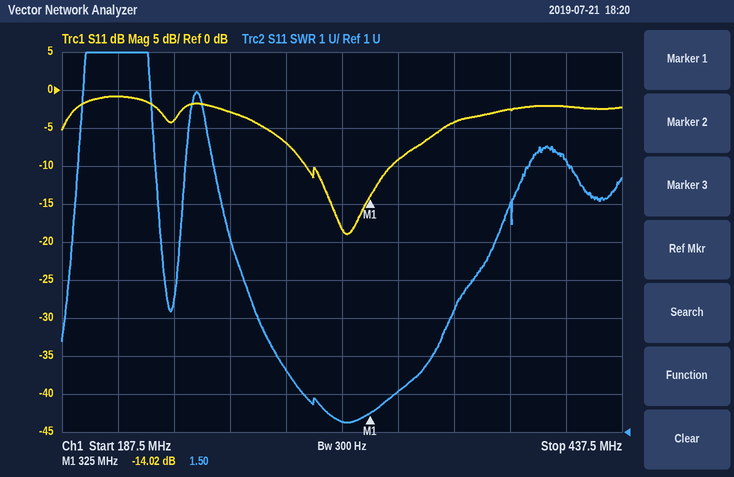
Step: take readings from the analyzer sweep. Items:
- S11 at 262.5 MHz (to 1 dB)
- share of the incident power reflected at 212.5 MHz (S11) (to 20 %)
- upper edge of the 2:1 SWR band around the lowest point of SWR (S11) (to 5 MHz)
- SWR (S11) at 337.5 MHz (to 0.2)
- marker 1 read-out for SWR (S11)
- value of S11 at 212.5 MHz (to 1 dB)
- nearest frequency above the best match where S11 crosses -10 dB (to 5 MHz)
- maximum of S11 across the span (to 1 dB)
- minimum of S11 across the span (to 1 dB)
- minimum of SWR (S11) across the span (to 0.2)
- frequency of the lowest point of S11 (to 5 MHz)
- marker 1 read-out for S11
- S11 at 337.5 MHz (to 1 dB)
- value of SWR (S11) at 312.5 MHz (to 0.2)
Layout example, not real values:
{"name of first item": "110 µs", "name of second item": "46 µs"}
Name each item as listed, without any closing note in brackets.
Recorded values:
{"S11 at 262.5 MHz": "-3 dB", "share of the incident power reflected at 212.5 MHz (S11)": "80 %", "upper edge of the 2:1 SWR band around the lowest point of SWR (S11)": "335 MHz", "SWR (S11) at 337.5 MHz": "2.0", "marker 1 read-out for SWR": "1.50", "value of S11 at 212.5 MHz": "-1 dB", "nearest frequency above the best match where S11 crosses -10 dB": "335 MHz", "maximum of S11 across the span": "-1 dB", "minimum of S11 across the span": "-19 dB", "minimum of SWR (S11) across the span": "1.2", "frequency of the lowest point of S11": "315 MHz", "marker 1 read-out for S11": "-14.02 dB", "S11 at 337.5 MHz": "-9 dB", "value of SWR (S11) at 312.5 MHz": "1.2"}
